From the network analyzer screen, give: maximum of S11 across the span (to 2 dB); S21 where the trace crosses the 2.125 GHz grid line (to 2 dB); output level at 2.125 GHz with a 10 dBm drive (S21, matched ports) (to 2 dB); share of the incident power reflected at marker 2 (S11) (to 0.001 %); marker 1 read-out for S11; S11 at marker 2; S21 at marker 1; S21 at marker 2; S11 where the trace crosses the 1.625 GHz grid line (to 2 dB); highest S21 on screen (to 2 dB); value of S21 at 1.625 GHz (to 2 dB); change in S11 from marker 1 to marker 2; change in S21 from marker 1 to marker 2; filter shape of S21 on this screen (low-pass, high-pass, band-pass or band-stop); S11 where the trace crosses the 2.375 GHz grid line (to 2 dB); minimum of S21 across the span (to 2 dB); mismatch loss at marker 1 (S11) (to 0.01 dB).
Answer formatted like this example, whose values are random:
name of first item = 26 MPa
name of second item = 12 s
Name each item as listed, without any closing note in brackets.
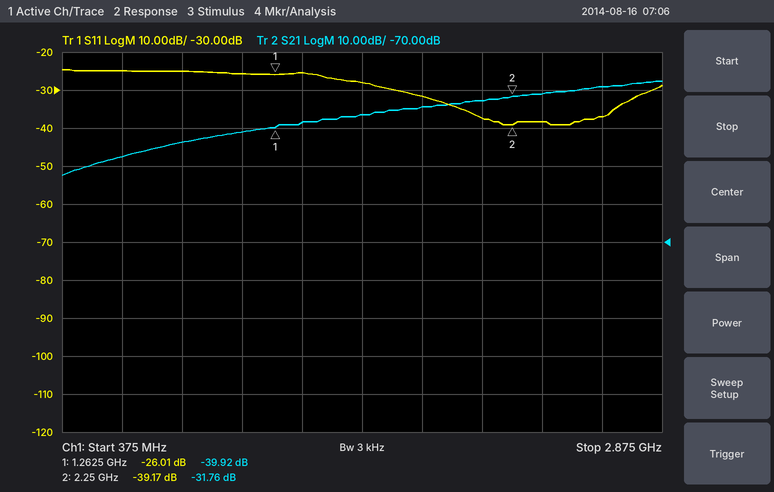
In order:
maximum of S11 across the span = -24 dB
S21 where the trace crosses the 2.125 GHz grid line = -32 dB
output level at 2.125 GHz with a 10 dBm drive (S21, matched ports) = -22 dBm
share of the incident power reflected at marker 2 (S11) = 0.012 %
marker 1 read-out for S11 = -26.01 dB
S11 at marker 2 = -39.17 dB
S21 at marker 1 = -39.92 dB
S21 at marker 2 = -31.76 dB
S11 where the trace crosses the 1.625 GHz grid line = -28 dB
highest S21 on screen = -28 dB
value of S21 at 1.625 GHz = -36 dB
change in S11 from marker 1 to marker 2 = -13.16 dB
change in S21 from marker 1 to marker 2 = 8.16 dB
filter shape of S21 on this screen = high-pass
S11 where the trace crosses the 2.375 GHz grid line = -38 dB
minimum of S21 across the span = -52 dB
mismatch loss at marker 1 (S11) = 0.01 dB
